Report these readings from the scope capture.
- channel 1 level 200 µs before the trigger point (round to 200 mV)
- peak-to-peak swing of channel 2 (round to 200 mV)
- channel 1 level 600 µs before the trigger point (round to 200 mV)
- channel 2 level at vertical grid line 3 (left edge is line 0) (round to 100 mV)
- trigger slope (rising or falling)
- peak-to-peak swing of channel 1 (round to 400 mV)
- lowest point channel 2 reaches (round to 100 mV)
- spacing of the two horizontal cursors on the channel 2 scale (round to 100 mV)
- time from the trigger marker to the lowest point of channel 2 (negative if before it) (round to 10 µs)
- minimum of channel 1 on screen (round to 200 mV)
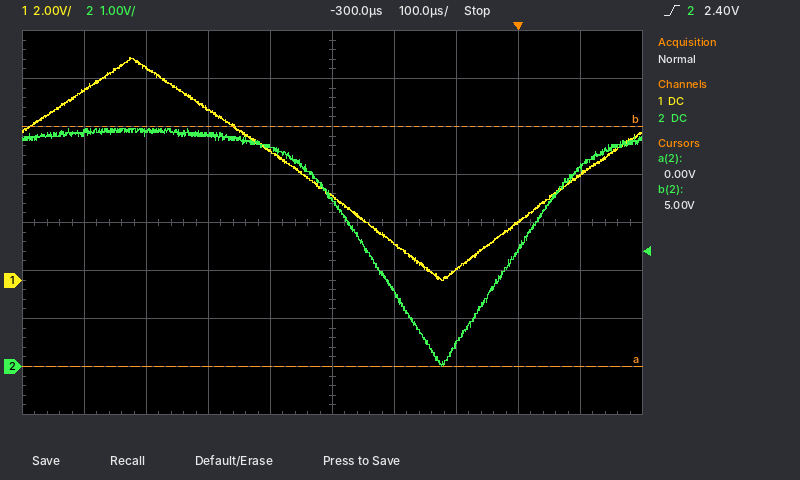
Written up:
1.6 V
5.0 V
8.8 V
4.8 V
rising
9.2 V
0.0 V
5.0 V
-120 µs
0.0 V
